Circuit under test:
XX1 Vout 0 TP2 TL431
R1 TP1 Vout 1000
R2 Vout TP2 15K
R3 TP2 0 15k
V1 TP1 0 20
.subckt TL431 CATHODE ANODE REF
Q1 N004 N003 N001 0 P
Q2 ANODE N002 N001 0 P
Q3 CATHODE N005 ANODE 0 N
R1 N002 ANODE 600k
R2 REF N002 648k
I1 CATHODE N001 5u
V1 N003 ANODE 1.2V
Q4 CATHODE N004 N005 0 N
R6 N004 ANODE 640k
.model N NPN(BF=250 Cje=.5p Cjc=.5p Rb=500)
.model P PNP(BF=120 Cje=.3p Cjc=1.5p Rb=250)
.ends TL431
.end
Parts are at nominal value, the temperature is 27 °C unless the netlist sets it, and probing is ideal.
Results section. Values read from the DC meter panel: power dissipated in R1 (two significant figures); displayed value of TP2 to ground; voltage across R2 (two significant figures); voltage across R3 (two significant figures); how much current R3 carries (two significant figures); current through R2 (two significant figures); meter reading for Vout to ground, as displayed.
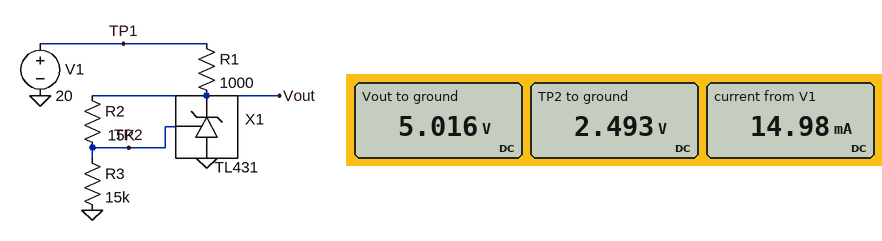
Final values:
220 mW
2.493 V
2.5 V
2.5 V
170 µA
170 µA
5.016 V
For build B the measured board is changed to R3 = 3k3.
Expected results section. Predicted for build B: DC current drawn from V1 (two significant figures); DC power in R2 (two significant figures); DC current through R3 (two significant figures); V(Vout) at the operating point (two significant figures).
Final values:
6.2 mA
8.5 mW
750 µA
14 V
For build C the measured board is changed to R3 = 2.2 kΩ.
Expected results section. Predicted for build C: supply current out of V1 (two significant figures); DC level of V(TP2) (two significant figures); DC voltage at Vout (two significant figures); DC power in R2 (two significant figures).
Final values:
1.1 mA
2.4 V
19 V
18 mW
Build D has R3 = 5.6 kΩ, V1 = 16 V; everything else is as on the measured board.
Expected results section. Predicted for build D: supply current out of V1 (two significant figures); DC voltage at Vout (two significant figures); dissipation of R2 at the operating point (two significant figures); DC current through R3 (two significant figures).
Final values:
6.8 mA
9.2 V
3.0 mW
440 µA
